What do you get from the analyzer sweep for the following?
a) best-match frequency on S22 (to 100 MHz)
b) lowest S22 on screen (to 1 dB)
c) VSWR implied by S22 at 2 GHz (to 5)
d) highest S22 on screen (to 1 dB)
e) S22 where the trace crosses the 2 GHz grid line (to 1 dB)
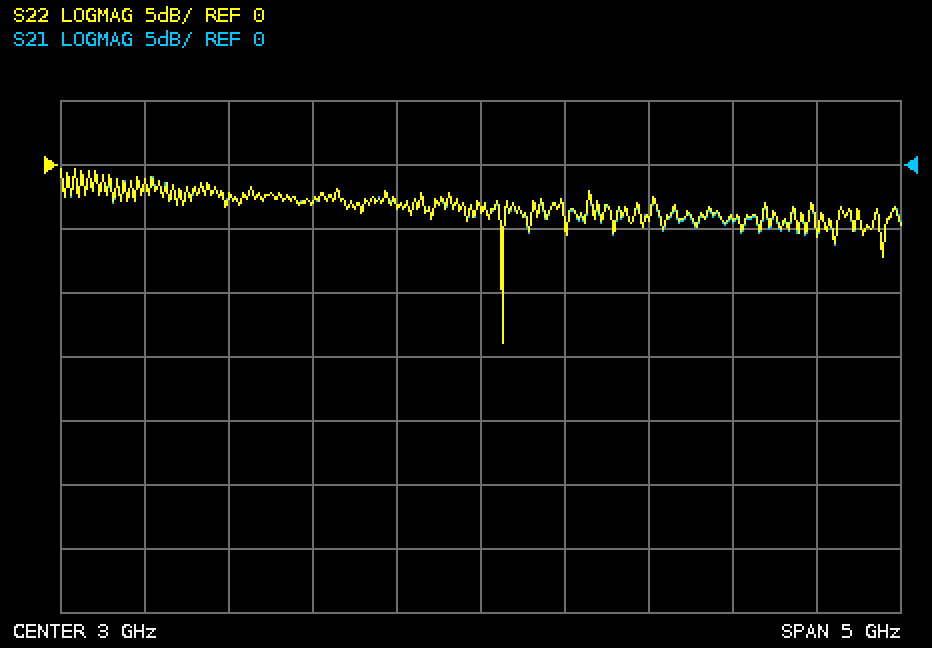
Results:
3.1 GHz
-14 dB
5
0 dB
-3 dB
